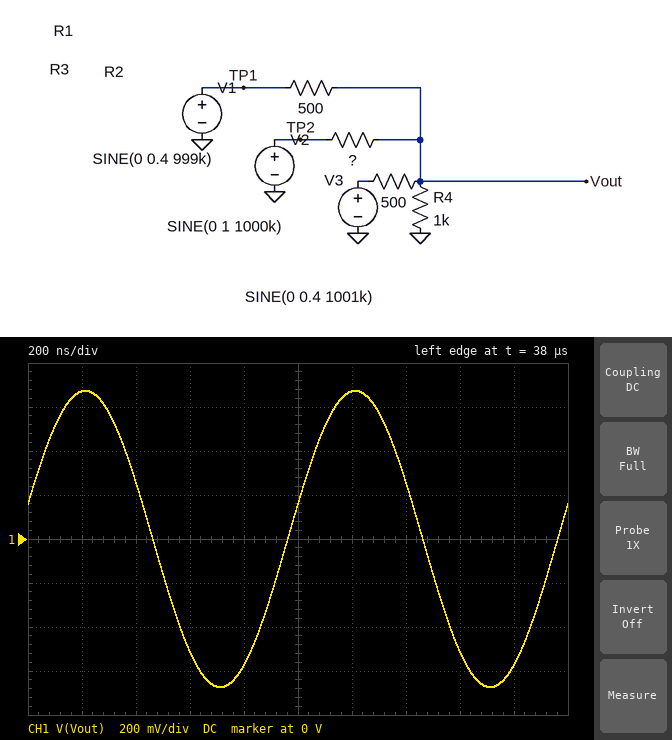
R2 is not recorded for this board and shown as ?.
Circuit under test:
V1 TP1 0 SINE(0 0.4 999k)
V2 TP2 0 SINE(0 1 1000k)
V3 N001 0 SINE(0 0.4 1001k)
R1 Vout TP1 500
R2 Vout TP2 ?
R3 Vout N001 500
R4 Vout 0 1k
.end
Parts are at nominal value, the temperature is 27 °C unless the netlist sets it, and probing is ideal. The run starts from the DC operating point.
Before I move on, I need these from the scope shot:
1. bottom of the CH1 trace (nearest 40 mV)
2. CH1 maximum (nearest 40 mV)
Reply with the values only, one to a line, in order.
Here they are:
-680 mV
680 mV
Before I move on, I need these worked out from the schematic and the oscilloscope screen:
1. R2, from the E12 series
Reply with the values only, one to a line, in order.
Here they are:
180 Ω
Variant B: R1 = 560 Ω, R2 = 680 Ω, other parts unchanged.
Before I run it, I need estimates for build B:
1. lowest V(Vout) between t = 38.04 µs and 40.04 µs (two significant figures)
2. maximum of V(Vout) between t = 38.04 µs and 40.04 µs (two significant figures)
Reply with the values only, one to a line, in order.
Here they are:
-470 mV
470 mV
